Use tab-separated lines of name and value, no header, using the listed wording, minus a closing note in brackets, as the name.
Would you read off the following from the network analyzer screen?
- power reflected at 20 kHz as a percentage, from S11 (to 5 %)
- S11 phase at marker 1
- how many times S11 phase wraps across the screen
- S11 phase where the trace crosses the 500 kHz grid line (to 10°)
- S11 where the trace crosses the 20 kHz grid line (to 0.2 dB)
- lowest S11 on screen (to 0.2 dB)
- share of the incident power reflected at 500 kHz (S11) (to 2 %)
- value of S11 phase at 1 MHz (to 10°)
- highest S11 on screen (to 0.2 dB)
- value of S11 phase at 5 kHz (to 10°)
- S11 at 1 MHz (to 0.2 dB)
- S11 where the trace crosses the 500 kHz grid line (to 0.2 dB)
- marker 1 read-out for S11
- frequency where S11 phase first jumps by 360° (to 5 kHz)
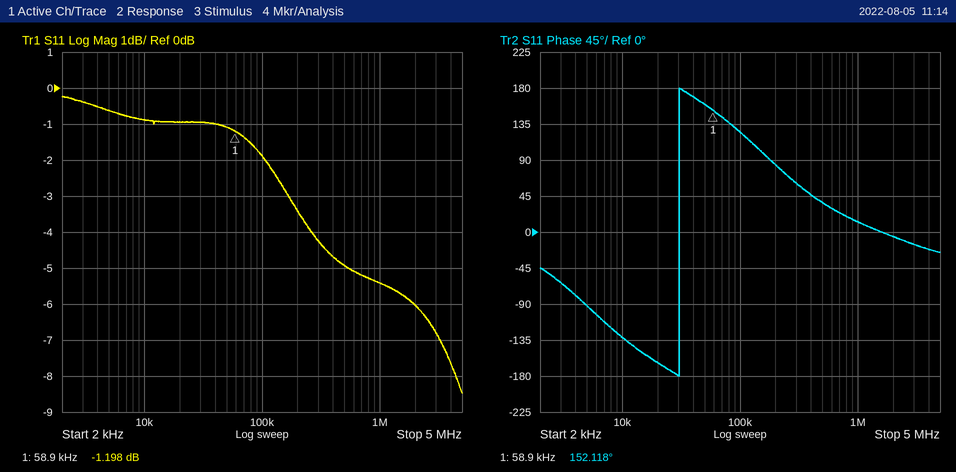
power reflected at 20 kHz as a percentage, from S11	80 %
S11 phase at marker 1	152.118°
how many times S11 phase wraps across the screen	1
S11 phase where the trace crosses the 500 kHz grid line	40°
S11 where the trace crosses the 20 kHz grid line	-1.0 dB
lowest S11 on screen	-8.4 dB
share of the incident power reflected at 500 kHz (S11)	32 %
value of S11 phase at 1 MHz	10°
highest S11 on screen	-0.2 dB
value of S11 phase at 5 kHz	-90°
S11 at 1 MHz	-5.4 dB
S11 where the trace crosses the 500 kHz grid line	-5.0 dB
marker 1 read-out for S11	-1.198 dB
frequency where S11 phase first jumps by 360°	30 kHz
